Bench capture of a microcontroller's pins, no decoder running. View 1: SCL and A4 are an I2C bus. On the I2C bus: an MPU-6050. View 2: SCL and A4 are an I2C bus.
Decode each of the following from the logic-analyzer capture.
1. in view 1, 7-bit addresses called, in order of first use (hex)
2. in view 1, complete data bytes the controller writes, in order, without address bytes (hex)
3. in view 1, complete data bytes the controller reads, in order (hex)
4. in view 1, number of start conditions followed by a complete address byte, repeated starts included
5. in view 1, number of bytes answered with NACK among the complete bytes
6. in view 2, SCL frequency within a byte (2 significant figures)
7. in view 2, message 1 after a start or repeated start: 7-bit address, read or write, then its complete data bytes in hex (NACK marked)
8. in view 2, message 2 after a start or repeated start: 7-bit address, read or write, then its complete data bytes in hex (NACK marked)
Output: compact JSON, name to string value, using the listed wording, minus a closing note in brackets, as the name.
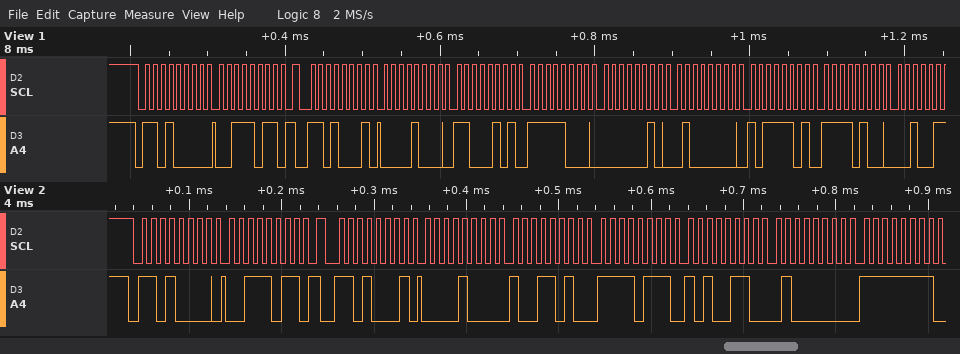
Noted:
{"in view 1, 7-bit addresses called, in order of first use": "0x68", "in view 1, complete data bytes the controller writes, in order, without address bytes": "3B", "in view 1, complete data bytes the controller reads, in order": "08 C5 F8 02 40 BD F4", "in view 1, number of start conditions followed by a complete address byte, repeated starts included": "2", "in view 1, number of bytes answered with NACK among the complete bytes": "0", "in view 2, SCL frequency within a byte": "100 kHz", "in view 2, message 1 after a start or repeated start: 7-bit address, read or write, then its complete data bytes in hex": "0x68 write: 3B", "in view 2, message 2 after a start or repeated start: 7-bit address, read or write, then its complete data bytes in hex": "0x68 read: 08 9A F7 A6 40 FF"}
